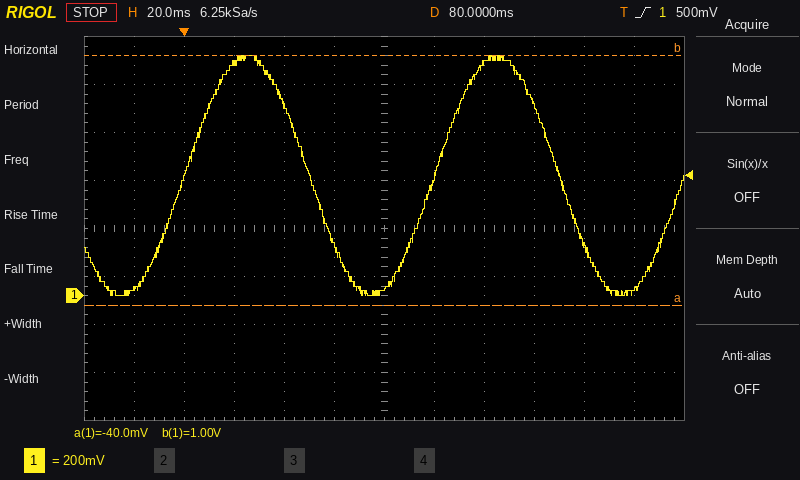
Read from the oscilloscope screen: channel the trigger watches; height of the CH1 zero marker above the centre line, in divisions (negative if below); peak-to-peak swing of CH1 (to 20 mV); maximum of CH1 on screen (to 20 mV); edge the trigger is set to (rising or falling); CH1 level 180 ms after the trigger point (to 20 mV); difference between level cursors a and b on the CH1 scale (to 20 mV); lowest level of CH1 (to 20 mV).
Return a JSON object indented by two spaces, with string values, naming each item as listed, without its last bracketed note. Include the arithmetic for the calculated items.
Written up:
{
  "channel the trigger watches": "CH1",
  "height of the CH1 zero marker above the centre line, in divisions": "-1.4 div",
  "peak-to-peak swing of CH1": "1.00 V − (0 mV) = 1.00 V",
  "maximum of CH1 on screen": "1.00 V",
  "edge the trigger is set to": "rising",
  "CH1 level 180 ms after the trigger point": "20 mV",
  "difference between level cursors a and b on the CH1 scale": "1.04 V",
  "lowest level of CH1": "0 mV"
}
